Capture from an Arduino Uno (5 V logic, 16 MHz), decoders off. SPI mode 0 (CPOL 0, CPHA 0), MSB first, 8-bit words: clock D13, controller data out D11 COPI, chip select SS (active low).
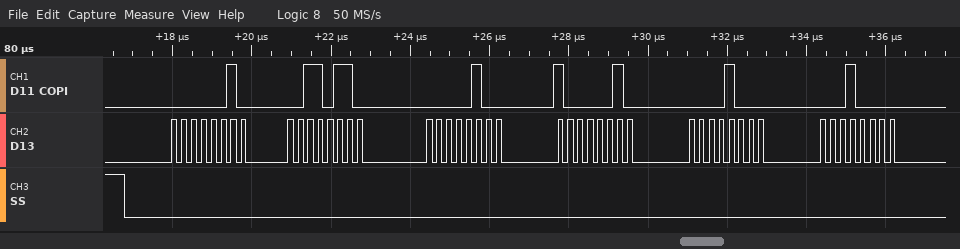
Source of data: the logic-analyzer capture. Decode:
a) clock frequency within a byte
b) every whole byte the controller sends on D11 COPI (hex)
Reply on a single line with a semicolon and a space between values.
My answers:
4 MHz; 02 36 04 82 08 10
